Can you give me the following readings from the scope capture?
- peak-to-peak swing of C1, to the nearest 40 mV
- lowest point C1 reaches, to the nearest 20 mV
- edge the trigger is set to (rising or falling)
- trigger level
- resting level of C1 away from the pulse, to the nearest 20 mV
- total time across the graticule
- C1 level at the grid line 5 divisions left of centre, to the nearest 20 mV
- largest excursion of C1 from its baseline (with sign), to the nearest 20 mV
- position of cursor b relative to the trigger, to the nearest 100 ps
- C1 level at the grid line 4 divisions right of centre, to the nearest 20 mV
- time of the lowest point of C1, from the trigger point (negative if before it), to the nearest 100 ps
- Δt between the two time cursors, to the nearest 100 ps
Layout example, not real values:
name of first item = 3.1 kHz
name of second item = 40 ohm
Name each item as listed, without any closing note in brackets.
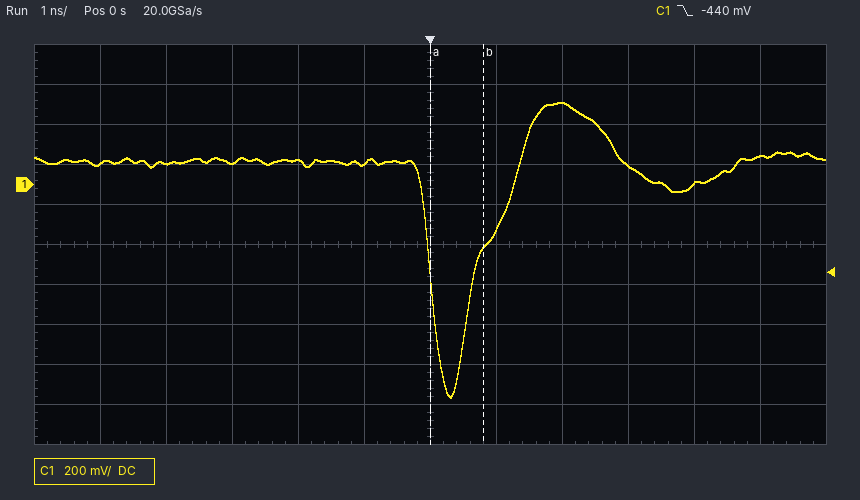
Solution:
peak-to-peak swing of C1, to the nearest 40 mV = 1.48 V
lowest point C1 reaches, to the nearest 20 mV = -1.06 V
edge the trigger is set to = falling
trigger level = -440 mV
resting level of C1 away from the pulse, to the nearest 20 mV = 120 mV
total time across the graticule = 12 ns
C1 level at the grid line 5 divisions left of centre, to the nearest 20 mV = 100 mV
largest excursion of C1 from its baseline (with sign), to the nearest 20 mV = -1.18 V
position of cursor b relative to the trigger, to the nearest 100 ps = +800 ps
C1 level at the grid line 4 divisions right of centre, to the nearest 20 mV = 0 mV
time of the lowest point of C1, from the trigger point (negative if before it), to the nearest 100 ps = +300 ps
Δt between the two time cursors, to the nearest 100 ps = 800 ps
